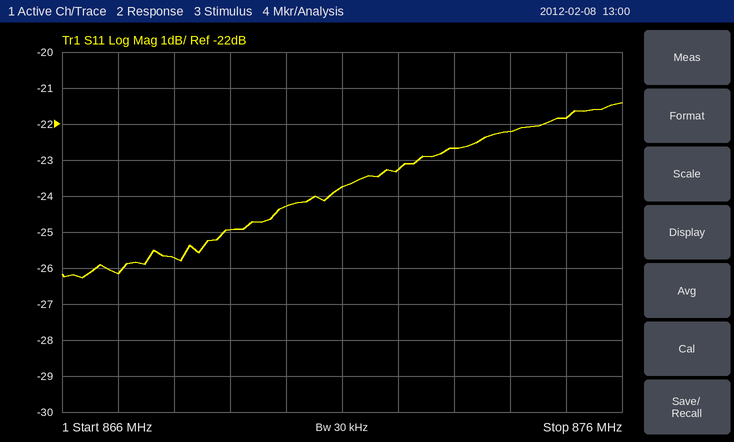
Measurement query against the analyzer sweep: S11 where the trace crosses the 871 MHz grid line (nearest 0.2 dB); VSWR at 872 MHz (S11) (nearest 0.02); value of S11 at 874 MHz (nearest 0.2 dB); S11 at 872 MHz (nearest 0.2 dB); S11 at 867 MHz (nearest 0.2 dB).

-23.8 dB
1.14
-22.2 dB
-23.2 dB
-26.2 dB
